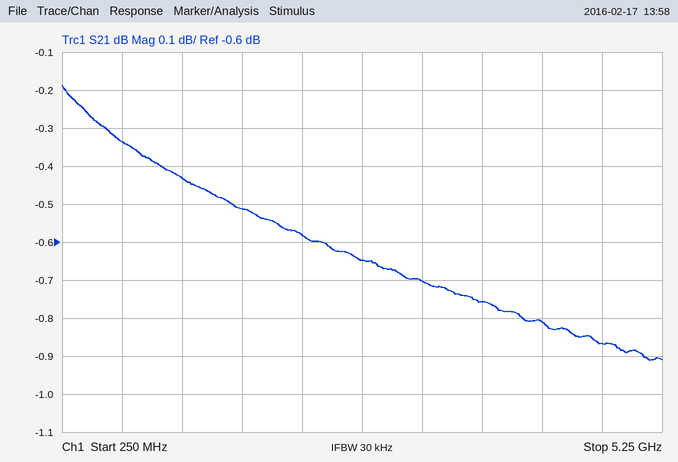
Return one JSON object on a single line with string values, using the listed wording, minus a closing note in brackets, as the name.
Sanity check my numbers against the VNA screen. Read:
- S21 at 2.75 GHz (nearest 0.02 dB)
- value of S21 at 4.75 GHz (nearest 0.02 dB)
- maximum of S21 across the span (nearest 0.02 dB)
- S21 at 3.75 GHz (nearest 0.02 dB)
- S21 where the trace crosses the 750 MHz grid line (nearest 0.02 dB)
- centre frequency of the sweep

{"S21 at 2.75 GHz": "-0.64 dB", "value of S21 at 4.75 GHz": "-0.86 dB", "maximum of S21 across the span": "-0.18 dB", "S21 at 3.75 GHz": "-0.76 dB", "S21 where the trace crosses the 750 MHz grid line": "-0.34 dB", "centre frequency of the sweep": "2.75 GHz"}
